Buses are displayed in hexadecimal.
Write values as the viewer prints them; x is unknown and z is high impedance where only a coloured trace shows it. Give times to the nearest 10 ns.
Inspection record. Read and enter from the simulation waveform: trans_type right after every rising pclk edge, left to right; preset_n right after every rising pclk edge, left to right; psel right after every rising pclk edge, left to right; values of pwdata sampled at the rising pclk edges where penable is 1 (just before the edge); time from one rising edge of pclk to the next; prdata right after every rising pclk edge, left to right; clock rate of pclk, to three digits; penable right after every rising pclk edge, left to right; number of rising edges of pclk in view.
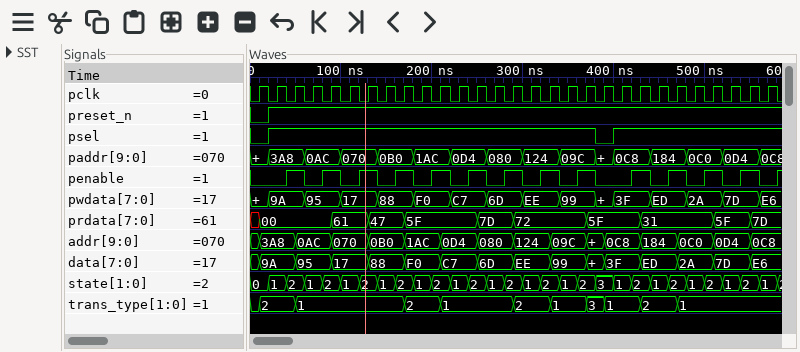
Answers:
2, 2, 1, 1, 1, 1, 1, 1, 2, 2, 1, 1, 1, 1, 2, 2, 1, 1, 3, 1, 1, 2, 2, 1, 1, 1, 1, 1, 1
0 1 1 1 1 1 1 1 1 1 1 1 1 1 1 1 1 1 1 1 1 1 1 1 1 1 1 1 1
0 1 1 1 1 1 1 1 1 1 1 1 1 1 1 1 1 1 1 0 1 1 1 1 1 1 1 1 1
9A, 95, 17, 88, F0, C7, 6D, EE, 99, 3F, ED, 2A, 7D
20 ns
00, 00, 00, 00, 61, 61, 47, 47, 5F, 5F, 5F, 5F, 7D, 7D, 72, 72, 72, 72, 5F, 5F, 5F, 31, 31, 31, 31, 5F, 5F, 7D, 7D
50.0 MHz
0 0 1 0 1 0 1 0 1 0 1 0 1 0 1 0 1 0 1 0 0 1 0 1 0 1 0 1 0
29
